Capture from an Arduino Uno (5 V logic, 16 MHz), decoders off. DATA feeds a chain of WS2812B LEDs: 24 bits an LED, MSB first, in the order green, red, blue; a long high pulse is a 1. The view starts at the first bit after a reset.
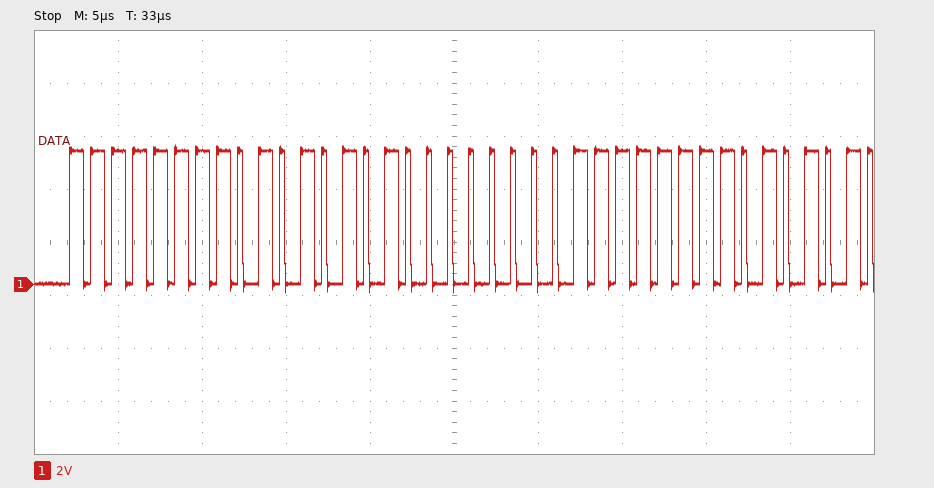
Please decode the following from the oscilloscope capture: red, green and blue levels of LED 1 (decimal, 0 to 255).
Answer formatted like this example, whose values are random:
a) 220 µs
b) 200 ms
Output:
a) 85, 255, 0
